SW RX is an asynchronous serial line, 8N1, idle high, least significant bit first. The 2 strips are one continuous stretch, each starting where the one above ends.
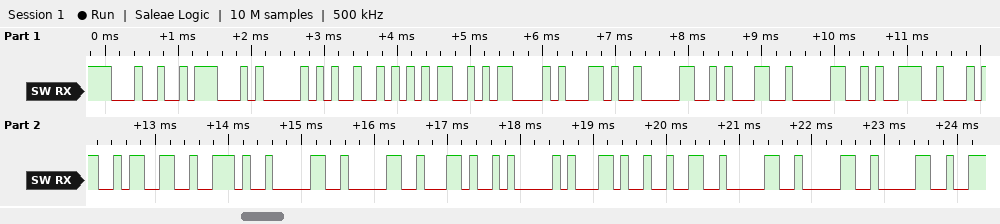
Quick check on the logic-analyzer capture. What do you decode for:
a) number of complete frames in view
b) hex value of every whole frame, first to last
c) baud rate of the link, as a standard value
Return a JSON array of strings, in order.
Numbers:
["23", "24 47 50 52 4D 43 2C 30 31 30 39 34 33 2E 30 30 2C 41 2C 32 30 30 30", "9600 baud"]
